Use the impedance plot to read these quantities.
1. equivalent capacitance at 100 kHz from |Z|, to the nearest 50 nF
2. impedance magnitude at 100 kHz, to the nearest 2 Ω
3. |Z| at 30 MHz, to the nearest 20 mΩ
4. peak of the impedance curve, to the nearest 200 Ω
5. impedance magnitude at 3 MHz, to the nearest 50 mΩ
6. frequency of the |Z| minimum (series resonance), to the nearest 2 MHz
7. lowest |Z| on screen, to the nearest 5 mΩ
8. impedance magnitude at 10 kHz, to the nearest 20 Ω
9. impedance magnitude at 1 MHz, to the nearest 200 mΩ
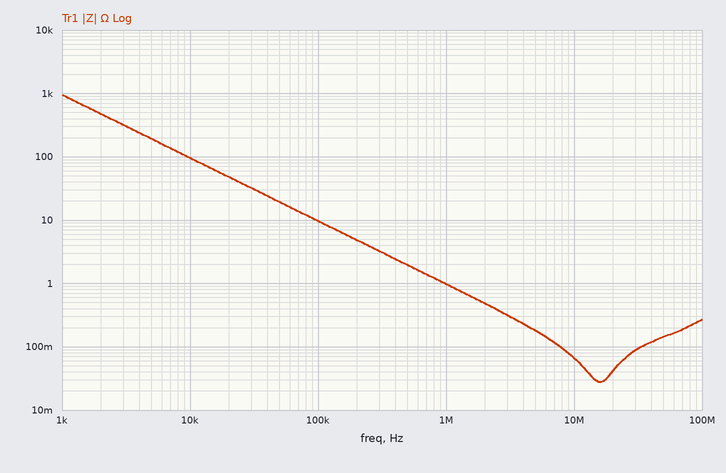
150 nF
10 Ω
80 mΩ
1.0 kΩ
300 mΩ
16 MHz
30 mΩ
100 Ω
1.0 Ω
